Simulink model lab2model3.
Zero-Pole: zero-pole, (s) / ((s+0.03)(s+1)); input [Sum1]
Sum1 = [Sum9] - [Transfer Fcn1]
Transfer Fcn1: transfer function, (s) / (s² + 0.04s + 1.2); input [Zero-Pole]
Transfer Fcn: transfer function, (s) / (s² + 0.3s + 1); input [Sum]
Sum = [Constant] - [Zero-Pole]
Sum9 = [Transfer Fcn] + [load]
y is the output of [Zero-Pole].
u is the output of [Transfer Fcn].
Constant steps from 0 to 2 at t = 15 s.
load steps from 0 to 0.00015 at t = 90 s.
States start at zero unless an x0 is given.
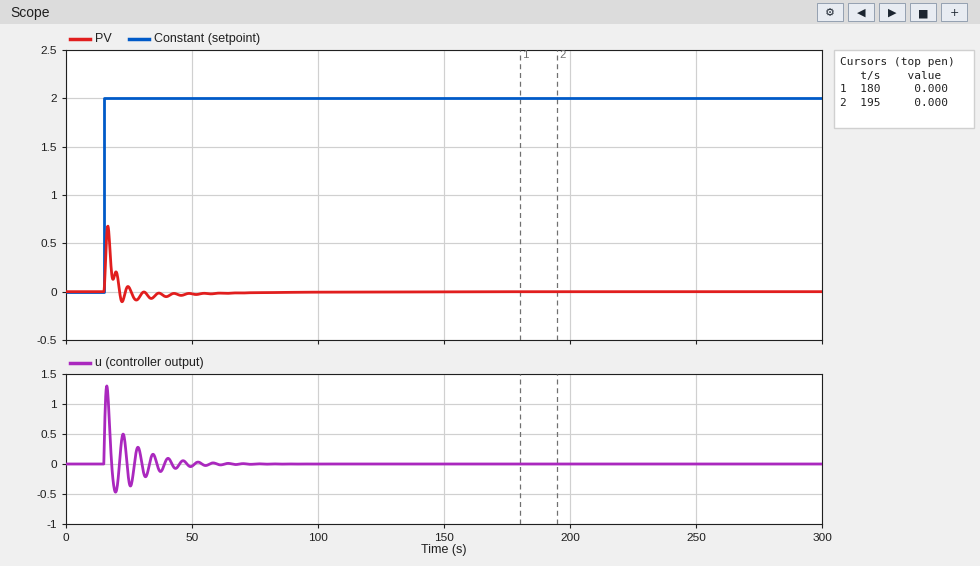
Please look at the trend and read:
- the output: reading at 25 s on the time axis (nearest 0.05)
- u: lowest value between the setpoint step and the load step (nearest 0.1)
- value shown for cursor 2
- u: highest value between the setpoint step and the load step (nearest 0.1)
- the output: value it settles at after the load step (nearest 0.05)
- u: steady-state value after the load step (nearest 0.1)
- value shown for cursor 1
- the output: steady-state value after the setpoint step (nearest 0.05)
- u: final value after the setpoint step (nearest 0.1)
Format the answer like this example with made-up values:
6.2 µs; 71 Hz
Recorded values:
0.05; -0.5; 0.000; 1.3; 0.00; 0.0; 0.000; 0.00; 0.0
